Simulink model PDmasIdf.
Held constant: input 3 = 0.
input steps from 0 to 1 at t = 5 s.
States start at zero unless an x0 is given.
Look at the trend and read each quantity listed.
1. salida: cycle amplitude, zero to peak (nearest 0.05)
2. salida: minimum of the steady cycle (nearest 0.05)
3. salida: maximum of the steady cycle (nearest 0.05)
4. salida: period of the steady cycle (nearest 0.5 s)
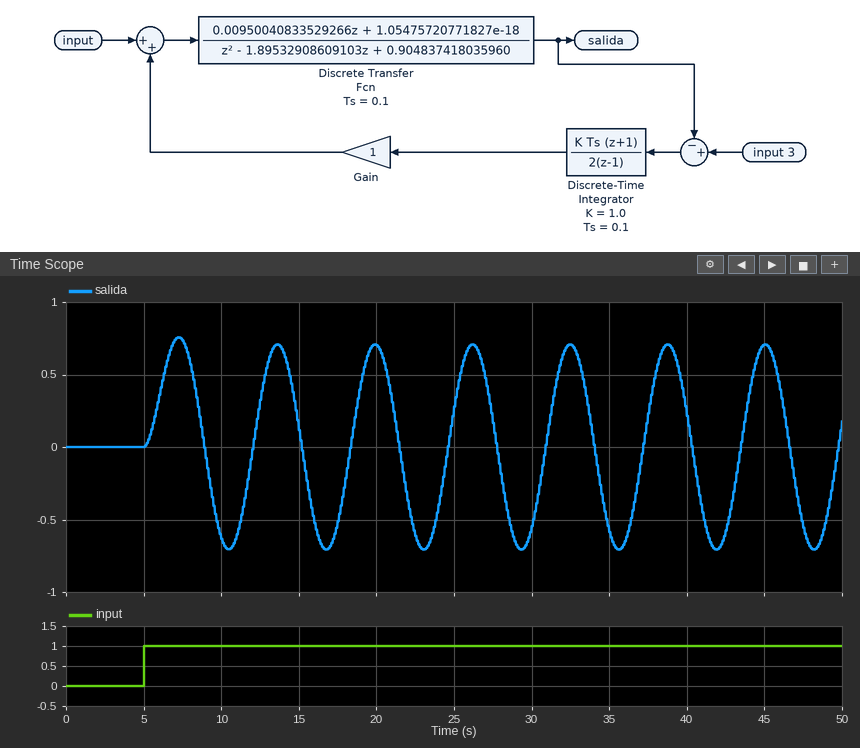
0.70
-0.70
0.70
6.5 s
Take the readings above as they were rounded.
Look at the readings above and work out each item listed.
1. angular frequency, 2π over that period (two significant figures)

0.97 rad/s
